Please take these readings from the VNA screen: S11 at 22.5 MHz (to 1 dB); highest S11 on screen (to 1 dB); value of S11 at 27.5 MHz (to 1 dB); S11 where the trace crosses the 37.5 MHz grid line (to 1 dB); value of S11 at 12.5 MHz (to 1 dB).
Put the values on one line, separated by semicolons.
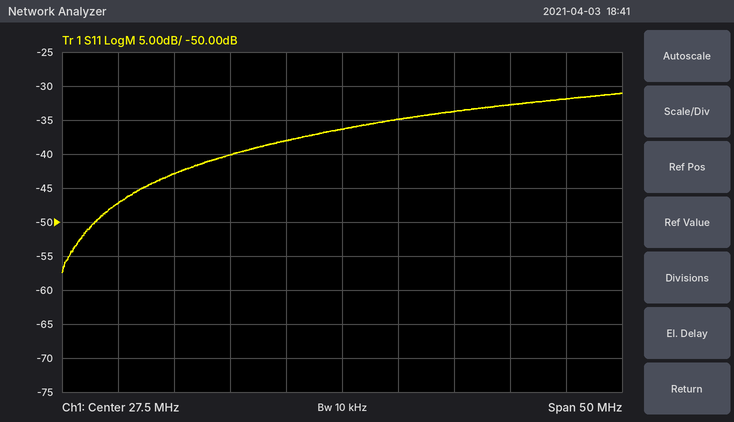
-38 dB; -31 dB; -36 dB; -34 dB; -43 dB
